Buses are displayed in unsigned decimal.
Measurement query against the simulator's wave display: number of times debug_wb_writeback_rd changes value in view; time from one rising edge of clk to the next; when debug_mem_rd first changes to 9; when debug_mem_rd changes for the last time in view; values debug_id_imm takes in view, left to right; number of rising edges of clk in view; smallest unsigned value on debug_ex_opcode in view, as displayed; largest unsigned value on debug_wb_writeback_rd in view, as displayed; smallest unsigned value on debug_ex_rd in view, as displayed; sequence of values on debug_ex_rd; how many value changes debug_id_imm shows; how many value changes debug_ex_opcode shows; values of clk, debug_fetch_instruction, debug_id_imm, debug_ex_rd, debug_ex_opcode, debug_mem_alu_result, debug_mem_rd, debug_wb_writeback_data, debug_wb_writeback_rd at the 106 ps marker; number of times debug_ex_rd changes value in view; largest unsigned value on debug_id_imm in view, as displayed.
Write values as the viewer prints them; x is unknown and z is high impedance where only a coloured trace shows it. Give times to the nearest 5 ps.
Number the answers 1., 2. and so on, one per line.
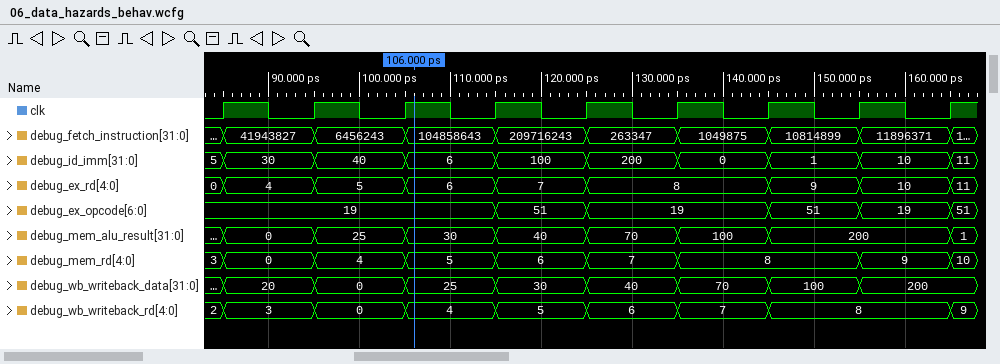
1. 8
2. 10 ps
3. 155 ps
4. 165 ps
5. 5, 30, 40, 6, 100, 200, 0, 1, 10, 11
6. 9
7. 19
8. 9
9. 0
10. 0, 4, 5, 6, 7, 8, 9, 10, 11
11. 9
12. 5
13. clk=1, debug_fetch_instruction=104858643, debug_id_imm=6, debug_ex_rd=6, debug_ex_opcode=19, debug_mem_alu_result=30, debug_mem_rd=5, debug_wb_writeback_data=25, debug_wb_writeback_rd=4
14. 8
15. 200
